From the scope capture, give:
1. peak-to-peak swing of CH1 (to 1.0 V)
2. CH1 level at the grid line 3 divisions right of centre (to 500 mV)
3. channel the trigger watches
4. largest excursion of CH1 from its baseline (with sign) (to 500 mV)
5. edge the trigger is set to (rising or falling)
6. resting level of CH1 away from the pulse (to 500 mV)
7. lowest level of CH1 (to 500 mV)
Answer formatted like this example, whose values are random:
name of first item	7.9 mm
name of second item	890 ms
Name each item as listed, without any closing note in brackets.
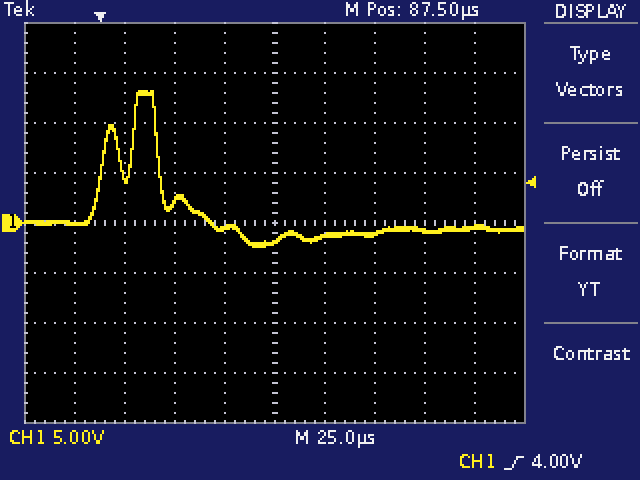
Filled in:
peak-to-peak swing of CH1	16.0 V
CH1 level at the grid line 3 divisions right of centre	-1.0 V
channel the trigger watches	CH1
largest excursion of CH1 from its baseline (with sign)	+14.0 V
edge the trigger is set to	rising
resting level of CH1 away from the pulse	-500 mV
lowest level of CH1	-2.5 V
